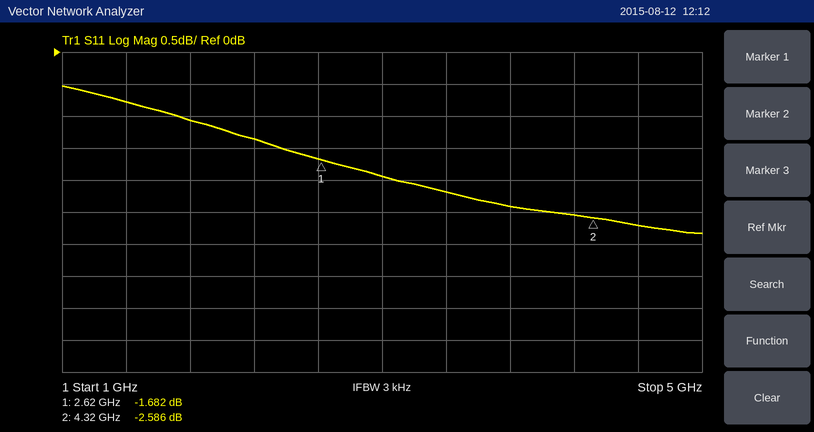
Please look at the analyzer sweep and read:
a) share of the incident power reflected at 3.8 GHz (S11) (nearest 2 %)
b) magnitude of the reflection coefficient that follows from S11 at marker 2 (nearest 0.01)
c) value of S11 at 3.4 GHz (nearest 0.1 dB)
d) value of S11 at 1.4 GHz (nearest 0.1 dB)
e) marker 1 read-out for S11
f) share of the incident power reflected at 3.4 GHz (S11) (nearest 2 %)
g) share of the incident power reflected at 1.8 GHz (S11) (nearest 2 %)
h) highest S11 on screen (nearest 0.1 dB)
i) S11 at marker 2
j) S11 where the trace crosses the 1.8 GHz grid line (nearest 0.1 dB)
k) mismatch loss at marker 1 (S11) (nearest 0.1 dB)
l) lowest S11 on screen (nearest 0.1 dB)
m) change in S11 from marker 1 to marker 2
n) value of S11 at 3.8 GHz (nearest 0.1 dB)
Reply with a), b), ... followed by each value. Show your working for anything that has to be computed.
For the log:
a) 10^(-2.4/10) ≈ 58 %
b) 10^(-2.586/20) ≈ 0.74
c) -2.2 dB
d) -0.8 dB
e) -1.682 dB
f) 10^(-2.2/10) ≈ 60 %
g) 10^(-1.1/10) ≈ 78 %
h) -0.5 dB
i) -2.586 dB
j) -1.1 dB
k) −10 log10(1 − 10^(-1.682/10)) ≈ 4.9 dB
l) -2.8 dB
m) -2.586 − (-1.682) = -0.904 dB
n) -2.4 dB
